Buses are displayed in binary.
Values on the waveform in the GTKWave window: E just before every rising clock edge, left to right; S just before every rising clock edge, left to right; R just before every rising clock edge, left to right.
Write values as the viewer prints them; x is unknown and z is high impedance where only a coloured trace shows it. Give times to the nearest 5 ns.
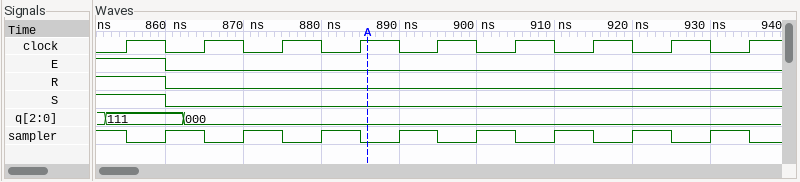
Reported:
1 0 0 0 0 0 0 0 0
1 0 0 0 0 0 0 0 0
1 0 0 0 0 0 0 0 0
